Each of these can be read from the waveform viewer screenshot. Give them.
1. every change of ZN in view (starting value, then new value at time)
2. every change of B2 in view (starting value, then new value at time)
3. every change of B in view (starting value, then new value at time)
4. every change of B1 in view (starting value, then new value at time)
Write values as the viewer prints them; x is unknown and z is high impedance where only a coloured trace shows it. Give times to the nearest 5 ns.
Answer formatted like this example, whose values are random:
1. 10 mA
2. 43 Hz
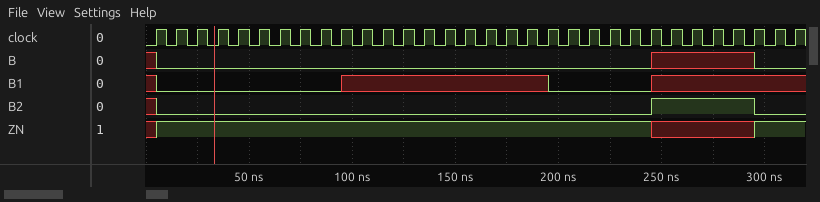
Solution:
1. x, 1 at 5 ns, x at 245 ns, 1 at 295 ns
2. x, 0 at 5 ns, 1 at 245 ns, 0 at 295 ns
3. x, 0 at 5 ns, x at 245 ns, 0 at 295 ns
4. x, 0 at 5 ns, x at 95 ns, 0 at 195 ns, x at 245 ns
